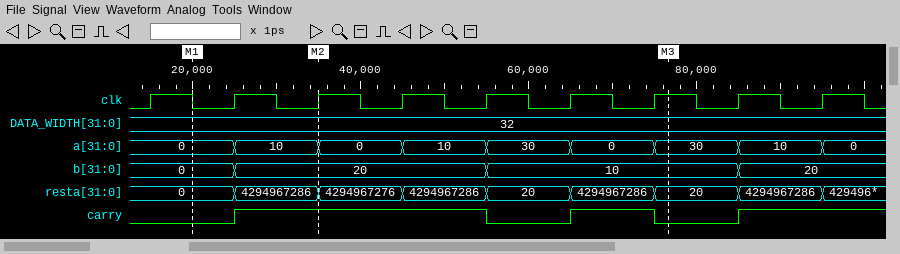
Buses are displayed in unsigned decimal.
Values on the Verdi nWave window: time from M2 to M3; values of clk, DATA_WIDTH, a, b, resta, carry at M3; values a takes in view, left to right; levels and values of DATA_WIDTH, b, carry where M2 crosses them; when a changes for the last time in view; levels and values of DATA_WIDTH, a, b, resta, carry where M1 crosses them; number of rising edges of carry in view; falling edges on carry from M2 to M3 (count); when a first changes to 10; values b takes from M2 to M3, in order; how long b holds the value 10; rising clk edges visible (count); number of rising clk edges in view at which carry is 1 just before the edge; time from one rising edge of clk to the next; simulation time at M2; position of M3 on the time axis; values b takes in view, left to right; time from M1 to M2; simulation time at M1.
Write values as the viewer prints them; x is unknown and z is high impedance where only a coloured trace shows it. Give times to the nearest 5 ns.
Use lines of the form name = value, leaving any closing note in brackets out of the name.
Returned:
time from M2 to M3 = 40 ns
values of clk, DATA_WIDTH, a, b, resta, carry at M3 = clk=1, DATA_WIDTH=32, a=30, b=10, resta=20, carry=0
values a takes in view, left to right = 0, 10, 0, 10, 30, 0, 30, 10, 0
levels and values of DATA_WIDTH, b, carry where M2 crosses them = DATA_WIDTH=32, b=20, carry=1
when a changes for the last time in view = 95 ns
levels and values of DATA_WIDTH, a, b, resta, carry where M1 crosses them = DATA_WIDTH=32, a=0, b=0, resta=0, carry=0
number of rising edges of carry in view = 3
falling edges on carry from M2 to M3 = 2
when a first changes to 10 = 25 ns
values b takes from M2 to M3, in order = 20, 10
how long b holds the value 10 = 30 ns
rising clk edges visible = 9
number of rising clk edges in view at which carry is 1 just before the edge = 5
time from one rising edge of clk to the next = 10 ns
simulation time at M2 = 35 ns
position of M3 on the time axis = 75 ns
values b takes in view, left to right = 0, 20, 10, 20
time from M1 to M2 = 15 ns
simulation time at M1 = 20 ns
